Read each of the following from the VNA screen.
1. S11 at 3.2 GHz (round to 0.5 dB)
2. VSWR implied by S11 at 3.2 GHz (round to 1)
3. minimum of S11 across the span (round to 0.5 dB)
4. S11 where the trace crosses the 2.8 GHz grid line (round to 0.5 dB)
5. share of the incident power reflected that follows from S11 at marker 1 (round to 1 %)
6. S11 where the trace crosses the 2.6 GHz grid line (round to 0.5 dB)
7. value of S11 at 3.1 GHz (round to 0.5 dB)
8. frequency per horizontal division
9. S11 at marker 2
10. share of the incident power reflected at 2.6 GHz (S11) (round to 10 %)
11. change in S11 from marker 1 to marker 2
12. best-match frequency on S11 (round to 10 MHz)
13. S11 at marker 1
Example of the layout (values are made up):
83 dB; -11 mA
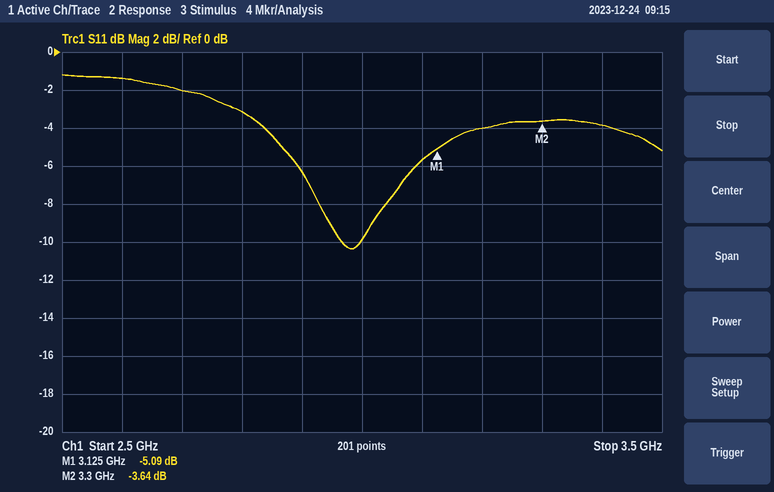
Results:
-4.0 dB; 4; -10.5 dB; -3.0 dB; 31 %; -1.5 dB; -5.5 dB; 100 MHz; -3.64 dB; 70 %; 1.45 dB; 2.98 GHz; -5.09 dB
